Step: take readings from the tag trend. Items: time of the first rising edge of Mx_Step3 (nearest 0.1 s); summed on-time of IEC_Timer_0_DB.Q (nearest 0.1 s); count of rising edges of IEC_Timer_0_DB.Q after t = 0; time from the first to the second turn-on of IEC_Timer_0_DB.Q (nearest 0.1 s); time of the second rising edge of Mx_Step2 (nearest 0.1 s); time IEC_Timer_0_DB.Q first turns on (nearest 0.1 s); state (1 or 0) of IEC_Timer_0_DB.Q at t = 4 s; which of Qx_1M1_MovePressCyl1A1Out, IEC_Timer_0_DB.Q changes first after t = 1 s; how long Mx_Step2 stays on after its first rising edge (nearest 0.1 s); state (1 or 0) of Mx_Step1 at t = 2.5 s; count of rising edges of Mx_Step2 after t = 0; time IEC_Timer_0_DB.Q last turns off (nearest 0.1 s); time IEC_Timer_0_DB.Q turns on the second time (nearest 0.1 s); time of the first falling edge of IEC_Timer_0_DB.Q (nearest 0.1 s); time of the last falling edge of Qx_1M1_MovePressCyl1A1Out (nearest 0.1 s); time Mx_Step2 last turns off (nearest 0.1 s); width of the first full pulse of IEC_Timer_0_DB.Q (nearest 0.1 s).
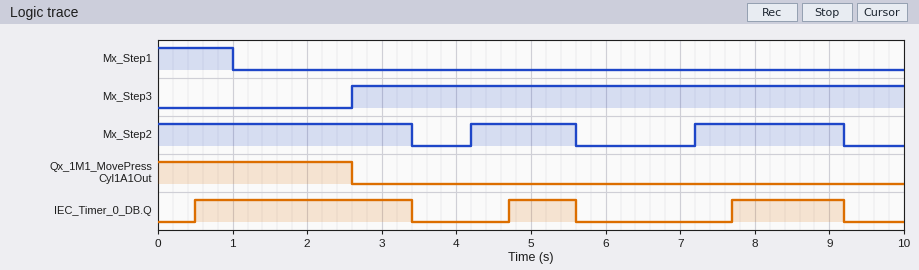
2.6 s
5.3 s
3
4.2 s
7.2 s
0.5 s
0
Qx_1M1_MovePressCyl1A1Out
1.4 s
0
2
9.2 s
4.7 s
3.4 s
2.6 s
9.2 s
2.9 s
